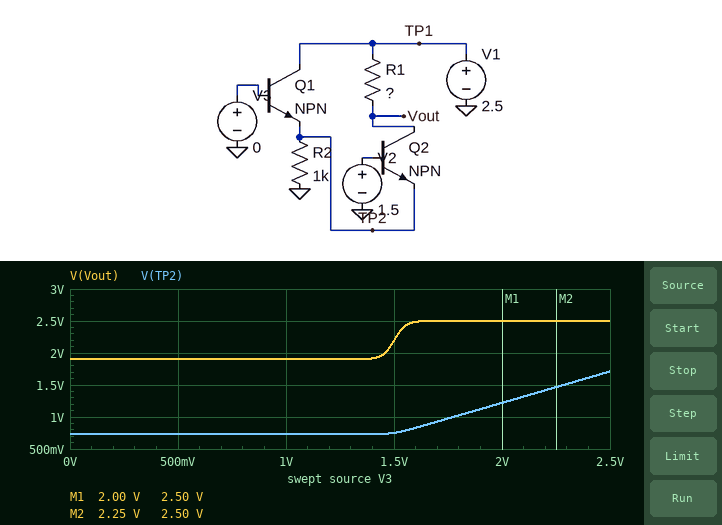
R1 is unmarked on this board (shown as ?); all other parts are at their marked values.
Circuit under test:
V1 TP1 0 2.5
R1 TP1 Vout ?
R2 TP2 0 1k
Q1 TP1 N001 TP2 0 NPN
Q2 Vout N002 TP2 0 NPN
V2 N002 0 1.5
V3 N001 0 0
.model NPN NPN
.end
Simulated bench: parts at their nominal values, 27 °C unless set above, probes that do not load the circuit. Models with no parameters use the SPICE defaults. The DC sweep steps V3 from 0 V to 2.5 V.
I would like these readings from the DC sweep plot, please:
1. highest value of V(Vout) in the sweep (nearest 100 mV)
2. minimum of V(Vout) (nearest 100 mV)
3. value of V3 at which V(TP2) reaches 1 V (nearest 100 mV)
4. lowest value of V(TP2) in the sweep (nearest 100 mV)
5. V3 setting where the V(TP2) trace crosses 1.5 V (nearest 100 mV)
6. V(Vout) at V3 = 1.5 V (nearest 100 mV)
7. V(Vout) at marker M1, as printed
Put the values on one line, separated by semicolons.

2.5 V; 1.9 V; 1.8 V; 700 mV; 2.3 V; 2.2 V; 2.50 V
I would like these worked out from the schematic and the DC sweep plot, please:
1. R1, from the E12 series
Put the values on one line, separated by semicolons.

820 Ω
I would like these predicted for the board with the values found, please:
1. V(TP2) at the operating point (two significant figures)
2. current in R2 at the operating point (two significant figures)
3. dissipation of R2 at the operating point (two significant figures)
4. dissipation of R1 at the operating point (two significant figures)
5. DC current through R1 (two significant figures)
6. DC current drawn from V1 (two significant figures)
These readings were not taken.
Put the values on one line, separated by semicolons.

730 mV; 730 µA; 540 µW; 430 µW; 730 µA; 730 µA
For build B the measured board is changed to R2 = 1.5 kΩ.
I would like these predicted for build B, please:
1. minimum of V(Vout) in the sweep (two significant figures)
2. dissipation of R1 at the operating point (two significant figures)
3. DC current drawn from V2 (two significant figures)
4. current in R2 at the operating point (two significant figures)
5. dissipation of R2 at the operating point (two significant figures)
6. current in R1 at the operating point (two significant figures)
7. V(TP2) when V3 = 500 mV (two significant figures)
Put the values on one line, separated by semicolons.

2.1 V; 200 µW; 4.9 µA; 500 µA; 370 µW; 490 µA; 740 mV
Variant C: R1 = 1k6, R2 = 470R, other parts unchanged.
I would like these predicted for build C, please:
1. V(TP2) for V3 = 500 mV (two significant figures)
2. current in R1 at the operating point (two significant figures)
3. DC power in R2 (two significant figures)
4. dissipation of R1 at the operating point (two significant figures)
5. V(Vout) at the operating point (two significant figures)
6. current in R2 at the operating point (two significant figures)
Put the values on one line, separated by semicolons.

710 mV; 1.1 mA; 1.1 mW; 1.9 mW; 750 mV; 1.5 mA
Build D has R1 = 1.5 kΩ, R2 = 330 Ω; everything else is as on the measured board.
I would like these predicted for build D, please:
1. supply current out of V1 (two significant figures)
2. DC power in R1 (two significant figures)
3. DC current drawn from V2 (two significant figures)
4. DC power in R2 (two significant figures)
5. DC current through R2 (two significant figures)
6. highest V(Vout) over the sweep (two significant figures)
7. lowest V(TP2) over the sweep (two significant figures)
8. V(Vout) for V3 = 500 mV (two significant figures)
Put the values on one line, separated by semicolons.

1.2 mA; 2.1 mW; 930 µA; 1.5 mW; 2.1 mA; 2.5 V; 700 mV; 730 mV
